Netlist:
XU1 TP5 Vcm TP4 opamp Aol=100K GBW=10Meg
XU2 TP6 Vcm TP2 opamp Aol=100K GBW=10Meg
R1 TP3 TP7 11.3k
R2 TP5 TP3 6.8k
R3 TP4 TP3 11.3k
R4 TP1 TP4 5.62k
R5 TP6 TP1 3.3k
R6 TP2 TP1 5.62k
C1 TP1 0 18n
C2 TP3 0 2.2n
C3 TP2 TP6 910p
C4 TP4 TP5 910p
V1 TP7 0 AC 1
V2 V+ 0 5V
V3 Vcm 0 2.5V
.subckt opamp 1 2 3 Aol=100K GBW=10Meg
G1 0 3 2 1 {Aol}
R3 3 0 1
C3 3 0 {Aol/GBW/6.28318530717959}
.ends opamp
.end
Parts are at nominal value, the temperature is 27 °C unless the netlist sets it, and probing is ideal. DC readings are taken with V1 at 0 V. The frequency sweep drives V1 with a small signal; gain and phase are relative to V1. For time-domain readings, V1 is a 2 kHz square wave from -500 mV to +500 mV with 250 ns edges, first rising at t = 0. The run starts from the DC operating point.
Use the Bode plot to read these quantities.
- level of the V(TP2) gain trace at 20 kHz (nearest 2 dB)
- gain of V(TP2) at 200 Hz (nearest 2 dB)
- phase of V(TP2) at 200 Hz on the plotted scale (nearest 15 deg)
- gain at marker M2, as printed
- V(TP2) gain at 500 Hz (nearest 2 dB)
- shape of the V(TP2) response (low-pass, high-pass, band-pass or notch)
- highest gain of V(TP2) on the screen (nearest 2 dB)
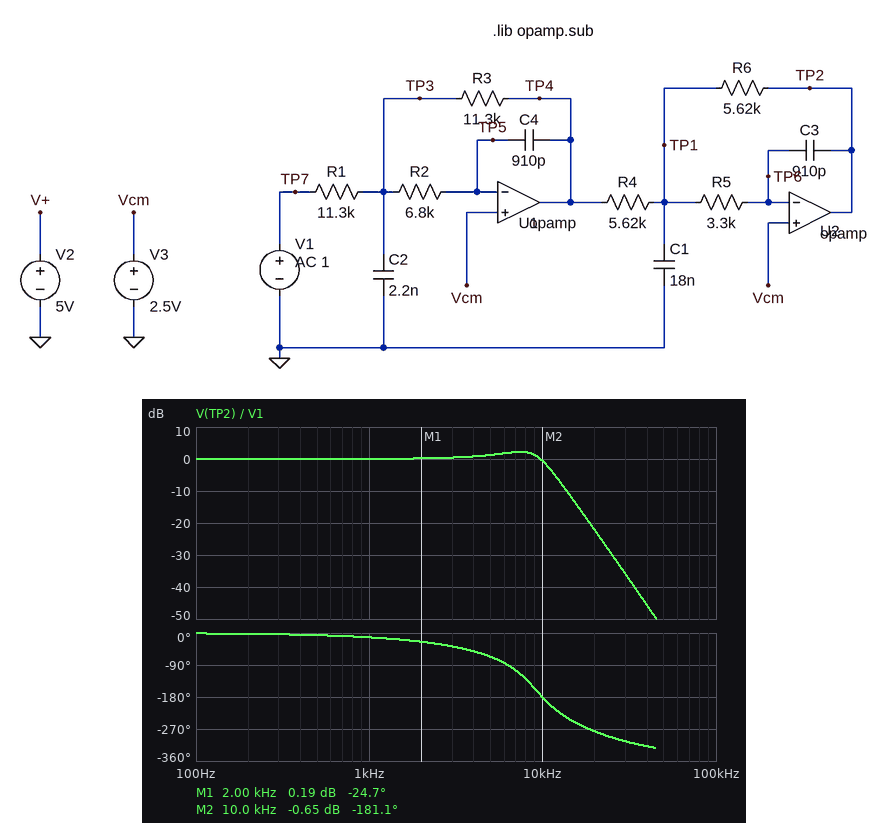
-22 dB
0 dB
0 deg
-0.65 dB
0 dB
low-pass
2 dB
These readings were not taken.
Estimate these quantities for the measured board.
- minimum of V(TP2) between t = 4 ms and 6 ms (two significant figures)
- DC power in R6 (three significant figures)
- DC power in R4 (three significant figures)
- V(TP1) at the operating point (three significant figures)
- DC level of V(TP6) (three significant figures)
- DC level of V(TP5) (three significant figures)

-730 mV
1.11 mW
1.11 mW
2.50 V
2.50 V
2.50 V
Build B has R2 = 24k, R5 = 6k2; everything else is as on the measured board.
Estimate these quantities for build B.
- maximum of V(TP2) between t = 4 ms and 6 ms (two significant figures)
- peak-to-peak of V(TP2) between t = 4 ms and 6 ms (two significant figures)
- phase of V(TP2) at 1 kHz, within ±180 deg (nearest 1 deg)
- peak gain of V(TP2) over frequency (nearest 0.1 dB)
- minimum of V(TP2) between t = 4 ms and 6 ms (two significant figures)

540 mV
1.1 V
-25 deg
0 dB
-540 mV
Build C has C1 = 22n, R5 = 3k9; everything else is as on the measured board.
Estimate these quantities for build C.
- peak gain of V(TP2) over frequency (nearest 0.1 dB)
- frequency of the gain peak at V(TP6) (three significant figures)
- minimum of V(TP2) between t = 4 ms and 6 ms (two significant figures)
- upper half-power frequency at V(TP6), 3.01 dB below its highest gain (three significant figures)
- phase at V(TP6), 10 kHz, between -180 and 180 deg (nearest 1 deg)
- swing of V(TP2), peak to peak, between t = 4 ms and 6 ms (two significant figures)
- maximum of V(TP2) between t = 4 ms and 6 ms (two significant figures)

3.5 dB
7.31 kHz
-790 mV
9.41 kHz
61 deg
1.6 V
790 mV
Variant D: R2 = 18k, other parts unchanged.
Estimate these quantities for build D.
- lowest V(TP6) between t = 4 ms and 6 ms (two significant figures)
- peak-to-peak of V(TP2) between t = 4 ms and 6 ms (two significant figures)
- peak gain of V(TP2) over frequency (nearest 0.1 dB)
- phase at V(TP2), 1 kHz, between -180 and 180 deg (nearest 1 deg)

2.5 V
1.1 V
0 dB
-19 deg
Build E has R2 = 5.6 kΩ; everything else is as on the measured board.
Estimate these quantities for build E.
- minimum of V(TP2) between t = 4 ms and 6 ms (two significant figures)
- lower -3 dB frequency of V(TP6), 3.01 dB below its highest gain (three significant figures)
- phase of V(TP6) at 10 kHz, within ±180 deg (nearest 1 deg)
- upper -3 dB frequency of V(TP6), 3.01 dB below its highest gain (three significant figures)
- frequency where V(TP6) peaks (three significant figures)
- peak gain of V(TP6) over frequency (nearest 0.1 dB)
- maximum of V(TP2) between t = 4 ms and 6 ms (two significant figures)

-750 mV
6.14 kHz
94 deg
11.3 kHz
8.67 kHz
-59.1 dB
750 mV
